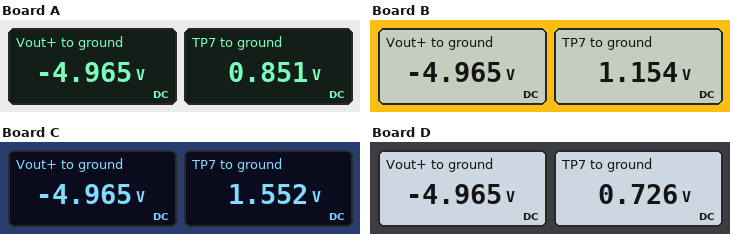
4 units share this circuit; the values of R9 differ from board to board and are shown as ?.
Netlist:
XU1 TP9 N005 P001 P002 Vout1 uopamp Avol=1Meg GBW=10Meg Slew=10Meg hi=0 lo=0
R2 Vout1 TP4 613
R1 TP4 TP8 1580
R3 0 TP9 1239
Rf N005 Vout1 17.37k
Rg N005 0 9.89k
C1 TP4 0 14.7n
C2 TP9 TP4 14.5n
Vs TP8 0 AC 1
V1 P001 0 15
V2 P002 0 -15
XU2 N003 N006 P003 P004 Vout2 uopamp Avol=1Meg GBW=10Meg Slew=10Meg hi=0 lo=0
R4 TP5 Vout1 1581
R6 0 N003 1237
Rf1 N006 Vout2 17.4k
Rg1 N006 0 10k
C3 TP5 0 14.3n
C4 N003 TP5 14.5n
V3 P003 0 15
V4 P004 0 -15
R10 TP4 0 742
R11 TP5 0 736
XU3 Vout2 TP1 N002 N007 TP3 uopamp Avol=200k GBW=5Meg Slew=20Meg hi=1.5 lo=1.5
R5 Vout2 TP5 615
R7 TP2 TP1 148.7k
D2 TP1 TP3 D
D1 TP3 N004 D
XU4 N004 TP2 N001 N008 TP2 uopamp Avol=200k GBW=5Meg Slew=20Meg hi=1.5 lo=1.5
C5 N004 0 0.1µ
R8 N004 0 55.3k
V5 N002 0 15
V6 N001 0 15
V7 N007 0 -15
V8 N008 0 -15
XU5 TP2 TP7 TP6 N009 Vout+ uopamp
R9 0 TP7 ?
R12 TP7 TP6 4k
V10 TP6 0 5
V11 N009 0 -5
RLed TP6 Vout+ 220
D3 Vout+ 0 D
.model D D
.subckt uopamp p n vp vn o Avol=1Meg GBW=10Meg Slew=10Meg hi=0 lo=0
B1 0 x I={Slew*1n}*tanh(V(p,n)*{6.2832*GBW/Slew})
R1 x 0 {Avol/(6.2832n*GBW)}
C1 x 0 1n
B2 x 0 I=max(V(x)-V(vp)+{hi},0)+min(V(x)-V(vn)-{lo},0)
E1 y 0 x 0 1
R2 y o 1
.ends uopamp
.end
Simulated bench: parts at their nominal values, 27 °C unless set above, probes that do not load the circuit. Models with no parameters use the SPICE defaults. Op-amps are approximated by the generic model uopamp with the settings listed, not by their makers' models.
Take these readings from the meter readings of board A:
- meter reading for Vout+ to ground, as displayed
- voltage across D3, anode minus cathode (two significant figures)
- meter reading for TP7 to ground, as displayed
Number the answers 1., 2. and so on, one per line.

1. -4.965 V
2. -5.0 V
3. 0.851 V
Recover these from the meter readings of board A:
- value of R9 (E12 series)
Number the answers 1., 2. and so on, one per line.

1. 820 Ω
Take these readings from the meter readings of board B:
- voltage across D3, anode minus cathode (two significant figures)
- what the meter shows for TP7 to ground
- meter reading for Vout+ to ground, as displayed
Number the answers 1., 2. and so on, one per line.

1. -5.0 V
2. 1.154 V
3. -4.965 V
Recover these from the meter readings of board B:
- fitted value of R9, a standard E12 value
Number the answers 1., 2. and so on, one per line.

1. 1.2 kΩ
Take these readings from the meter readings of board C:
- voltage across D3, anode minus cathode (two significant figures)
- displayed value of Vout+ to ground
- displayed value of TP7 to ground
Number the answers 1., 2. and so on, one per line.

1. -5.0 V
2. -4.965 V
3. 1.552 V
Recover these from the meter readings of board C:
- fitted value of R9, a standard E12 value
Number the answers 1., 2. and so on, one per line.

1. 1.8 kΩ
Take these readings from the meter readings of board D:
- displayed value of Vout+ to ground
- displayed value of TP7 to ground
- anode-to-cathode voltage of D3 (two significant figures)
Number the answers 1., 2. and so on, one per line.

1. -4.965 V
2. 0.726 V
3. -5.0 V
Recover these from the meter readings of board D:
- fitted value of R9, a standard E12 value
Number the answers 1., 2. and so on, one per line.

1. 680 Ω
